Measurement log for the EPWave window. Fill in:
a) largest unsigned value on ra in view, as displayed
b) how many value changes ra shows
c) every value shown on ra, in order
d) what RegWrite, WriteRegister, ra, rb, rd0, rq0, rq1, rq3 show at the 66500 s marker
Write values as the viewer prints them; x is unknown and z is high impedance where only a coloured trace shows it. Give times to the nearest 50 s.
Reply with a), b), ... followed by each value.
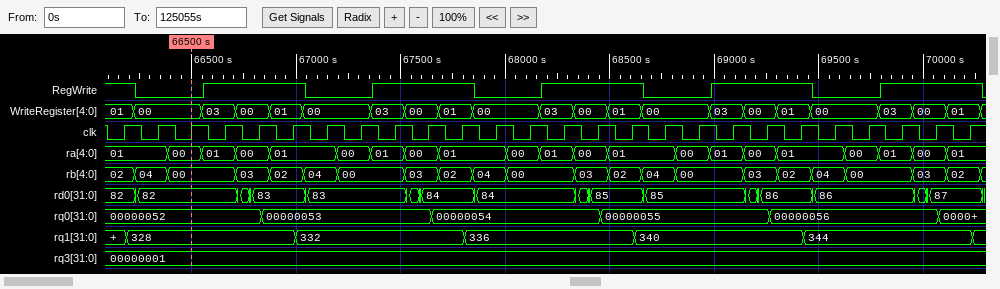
a) 01
b) 20
c) 01, 00, 01, 00, 01, 00, 01, 00, 01, 00, 01, 00, 01, 00, 01, 00, 01, 00, 01, 00, 01
d) RegWrite=0, WriteRegister=00, ra=00, rb=00, rd0=82, rq0=00000052, rq1=328, rq3=00000001
